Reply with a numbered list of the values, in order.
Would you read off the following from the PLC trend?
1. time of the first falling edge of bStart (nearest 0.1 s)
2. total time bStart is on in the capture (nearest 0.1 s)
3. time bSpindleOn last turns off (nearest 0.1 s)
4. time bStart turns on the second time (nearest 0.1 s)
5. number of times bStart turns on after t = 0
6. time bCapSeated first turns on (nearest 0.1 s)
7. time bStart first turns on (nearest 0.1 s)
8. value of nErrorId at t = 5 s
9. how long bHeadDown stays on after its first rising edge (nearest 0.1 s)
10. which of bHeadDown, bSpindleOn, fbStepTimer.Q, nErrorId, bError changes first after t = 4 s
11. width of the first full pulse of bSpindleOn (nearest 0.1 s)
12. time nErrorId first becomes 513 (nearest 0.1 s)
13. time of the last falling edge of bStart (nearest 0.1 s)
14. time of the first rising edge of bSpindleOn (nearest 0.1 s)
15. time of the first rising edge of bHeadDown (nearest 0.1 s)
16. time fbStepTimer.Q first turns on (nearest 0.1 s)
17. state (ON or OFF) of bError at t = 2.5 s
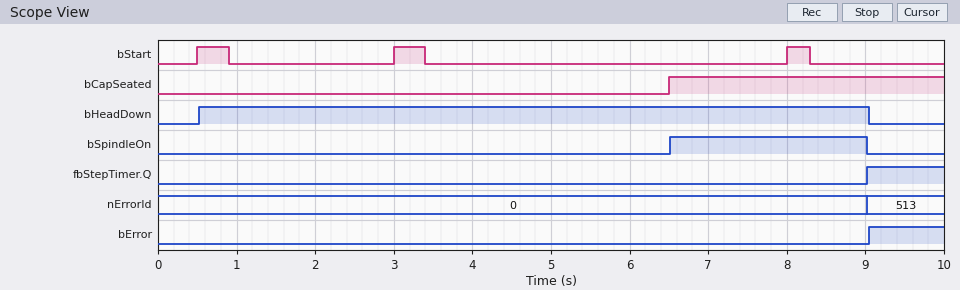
1. 0.9 s
2. 1.1 s
3. 9.0 s
4. 3.0 s
5. 3
6. 6.5 s
7. 0.5 s
8. 0
9. 8.5 s
10. bSpindleOn
11. 2.5 s
12. 9.0 s
13. 8.3 s
14. 6.5 s
15. 0.5 s
16. 9.0 s
17. OFF
